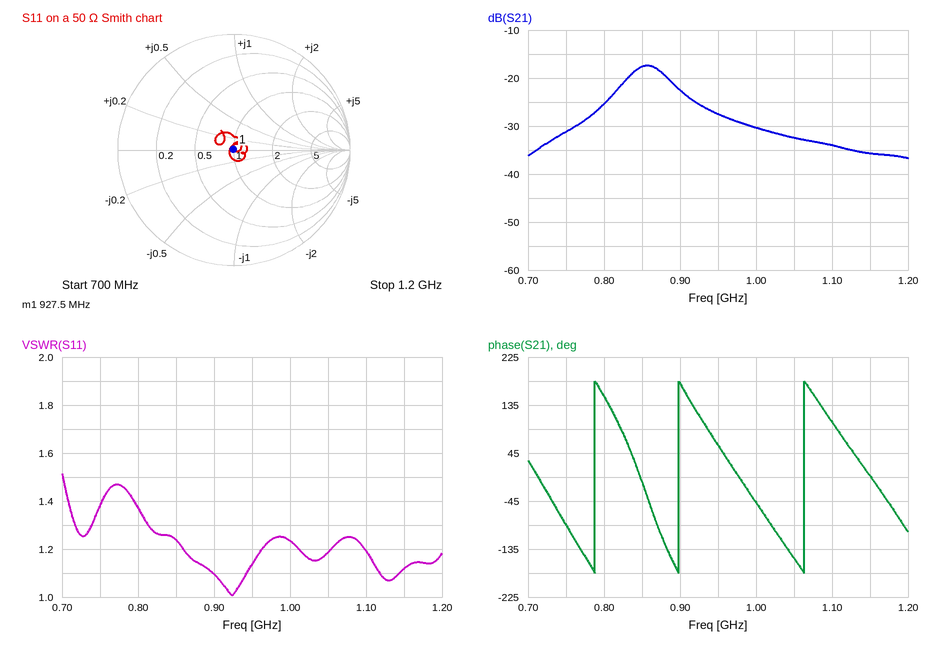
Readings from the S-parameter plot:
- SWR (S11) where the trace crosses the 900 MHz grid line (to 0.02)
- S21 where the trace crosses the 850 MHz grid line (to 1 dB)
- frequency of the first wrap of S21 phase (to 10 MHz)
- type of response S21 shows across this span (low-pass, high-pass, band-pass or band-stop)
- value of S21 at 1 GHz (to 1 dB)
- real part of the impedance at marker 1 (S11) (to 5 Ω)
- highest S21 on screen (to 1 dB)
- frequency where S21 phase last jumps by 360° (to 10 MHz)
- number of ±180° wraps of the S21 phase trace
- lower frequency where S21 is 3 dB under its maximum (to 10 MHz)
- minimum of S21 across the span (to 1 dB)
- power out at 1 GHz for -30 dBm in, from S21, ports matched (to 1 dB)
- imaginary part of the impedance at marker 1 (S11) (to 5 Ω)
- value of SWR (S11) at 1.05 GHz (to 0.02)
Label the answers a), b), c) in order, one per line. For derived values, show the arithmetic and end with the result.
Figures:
a) 1.10
b) -18 dB
c) 790 MHz
d) band-pass
e) -30 dB
f) 50 Ω
g) -17 dB
h) 1.06 GHz
i) 3
j) 830 MHz
k) -37 dB
l) -30 dBm + (-30 dB) = -60 dBm
m) 0 Ω
n) 1.18
